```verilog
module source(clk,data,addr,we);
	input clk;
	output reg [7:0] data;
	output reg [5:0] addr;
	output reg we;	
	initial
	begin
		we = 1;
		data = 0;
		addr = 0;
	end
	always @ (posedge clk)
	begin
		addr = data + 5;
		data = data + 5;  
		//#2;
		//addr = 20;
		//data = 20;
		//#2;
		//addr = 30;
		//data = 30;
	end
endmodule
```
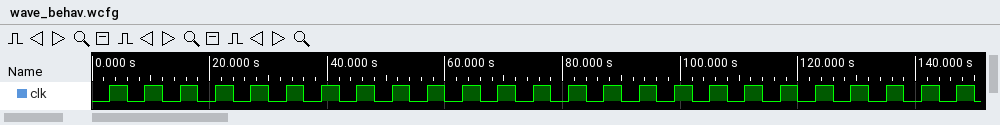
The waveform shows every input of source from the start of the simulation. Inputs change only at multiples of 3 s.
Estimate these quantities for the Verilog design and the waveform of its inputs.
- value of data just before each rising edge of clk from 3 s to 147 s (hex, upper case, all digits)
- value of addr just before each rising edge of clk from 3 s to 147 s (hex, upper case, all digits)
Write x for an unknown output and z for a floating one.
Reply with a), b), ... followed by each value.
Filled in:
a) 00, 05, 0A, 0F, 14, 19, 1E, 23, 28, 2D, 32, 37, 3C, 41, 46, 4B, 50, 55, 5A, 5F, 64, 69, 6E, 73, 78
b) 00, 05, 0A, 0F, 14, 19, 1E, 23, 28, 2D, 32, 37, 3C, 01, 06, 0B, 10, 15, 1A, 1F, 24, 29, 2E, 33, 38
